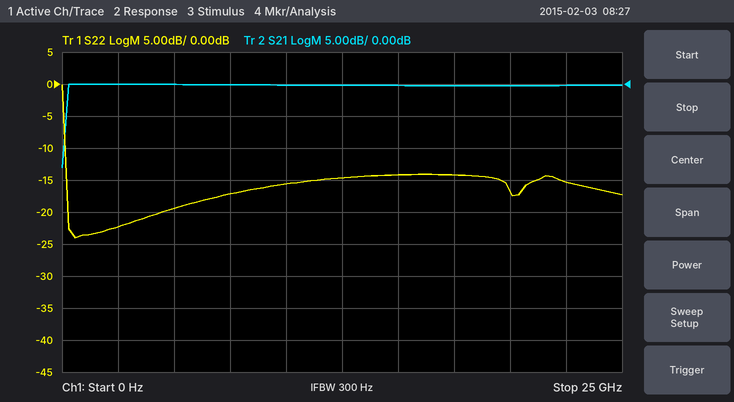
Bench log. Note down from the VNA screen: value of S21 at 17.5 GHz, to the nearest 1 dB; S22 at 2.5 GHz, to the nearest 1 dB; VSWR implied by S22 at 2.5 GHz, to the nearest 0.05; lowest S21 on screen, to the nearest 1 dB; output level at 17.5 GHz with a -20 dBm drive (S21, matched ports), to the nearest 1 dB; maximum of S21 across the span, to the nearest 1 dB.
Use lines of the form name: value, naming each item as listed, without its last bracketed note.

value of S21 at 17.5 GHz, to the nearest 1 dB: 0 dB
S22 at 2.5 GHz, to the nearest 1 dB: -22 dB
VSWR implied by S22 at 2.5 GHz, to the nearest 0.05: 1.15
lowest S21 on screen, to the nearest 1 dB: -13 dB
output level at 17.5 GHz with a -20 dBm drive (S21, matched ports), to the nearest 1 dB: -20 dBm
maximum of S21 across the span, to the nearest 1 dB: 0 dB
